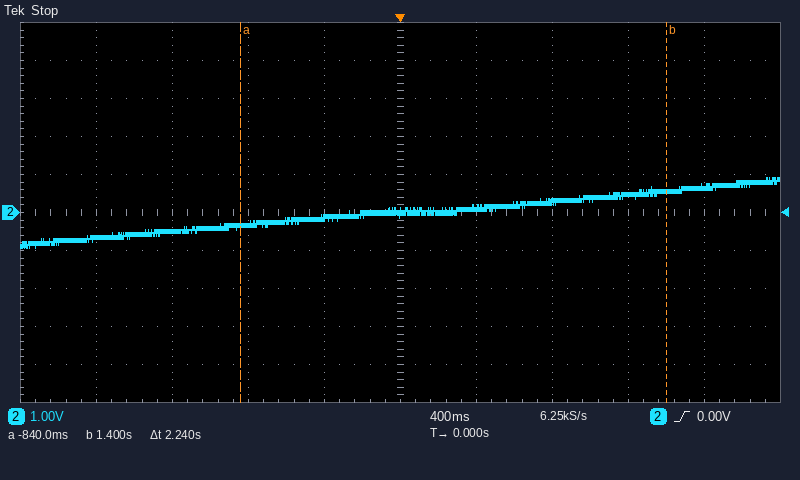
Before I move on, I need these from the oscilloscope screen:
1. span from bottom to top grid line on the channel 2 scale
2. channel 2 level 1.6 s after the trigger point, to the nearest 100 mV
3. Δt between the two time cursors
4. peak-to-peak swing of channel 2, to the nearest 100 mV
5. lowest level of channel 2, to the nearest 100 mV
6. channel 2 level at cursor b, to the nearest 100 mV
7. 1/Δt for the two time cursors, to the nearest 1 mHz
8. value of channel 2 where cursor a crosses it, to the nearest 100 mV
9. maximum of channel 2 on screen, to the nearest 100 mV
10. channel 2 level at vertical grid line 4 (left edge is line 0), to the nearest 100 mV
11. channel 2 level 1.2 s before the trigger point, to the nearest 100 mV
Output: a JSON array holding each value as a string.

["10 V", "700 mV", "2.24 s", "1.8 V", "-900 mV", "600 mV", "446 mHz", "-300 mV", "900 mV", "-100 mV", "-500 mV"]
